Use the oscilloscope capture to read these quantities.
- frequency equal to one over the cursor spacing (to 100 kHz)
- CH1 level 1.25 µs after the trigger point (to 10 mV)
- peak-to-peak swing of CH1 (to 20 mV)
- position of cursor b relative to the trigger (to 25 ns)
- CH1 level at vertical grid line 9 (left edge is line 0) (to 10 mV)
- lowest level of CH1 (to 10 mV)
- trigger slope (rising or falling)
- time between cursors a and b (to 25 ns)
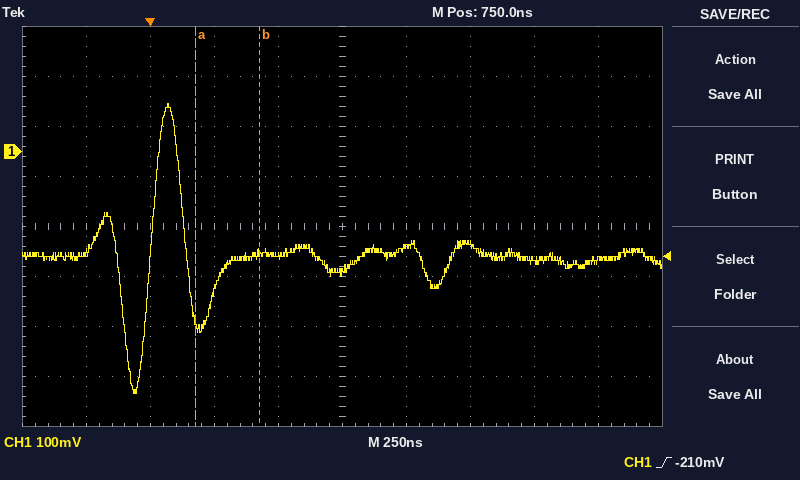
4.0 MHz
-190 mV
580 mV
+425 ns
-220 mV
-480 mV
rising
250 ns
